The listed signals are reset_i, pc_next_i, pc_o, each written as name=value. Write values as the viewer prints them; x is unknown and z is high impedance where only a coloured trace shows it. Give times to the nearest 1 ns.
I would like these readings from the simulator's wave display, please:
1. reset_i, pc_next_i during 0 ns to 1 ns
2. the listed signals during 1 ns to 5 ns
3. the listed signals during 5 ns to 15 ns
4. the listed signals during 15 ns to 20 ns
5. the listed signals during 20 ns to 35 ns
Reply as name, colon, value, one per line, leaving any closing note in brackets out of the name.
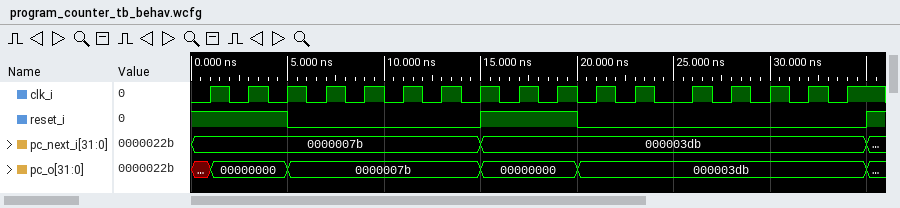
reset_i, pc_next_i during 0 ns to 1 ns: reset_i=1, pc_next_i=0000007b
the listed signals during 1 ns to 5 ns: reset_i=1, pc_next_i=0000007b, pc_o=00000000
the listed signals during 5 ns to 15 ns: reset_i=0, pc_next_i=0000007b, pc_o=0000007b
the listed signals during 15 ns to 20 ns: reset_i=1, pc_next_i=000003db, pc_o=00000000
the listed signals during 20 ns to 35 ns: reset_i=0, pc_next_i=000003db, pc_o=000003db
